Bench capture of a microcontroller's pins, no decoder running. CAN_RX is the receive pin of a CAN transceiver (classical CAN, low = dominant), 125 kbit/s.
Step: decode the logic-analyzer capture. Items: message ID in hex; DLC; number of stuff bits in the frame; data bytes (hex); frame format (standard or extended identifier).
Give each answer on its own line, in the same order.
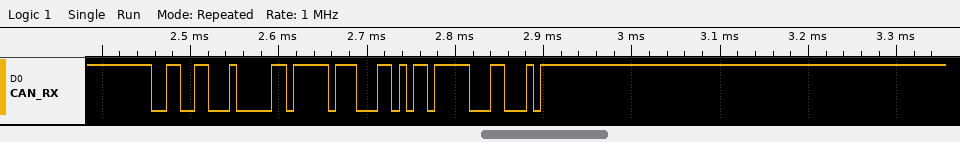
0x331
2
3
FF 1A
standard
